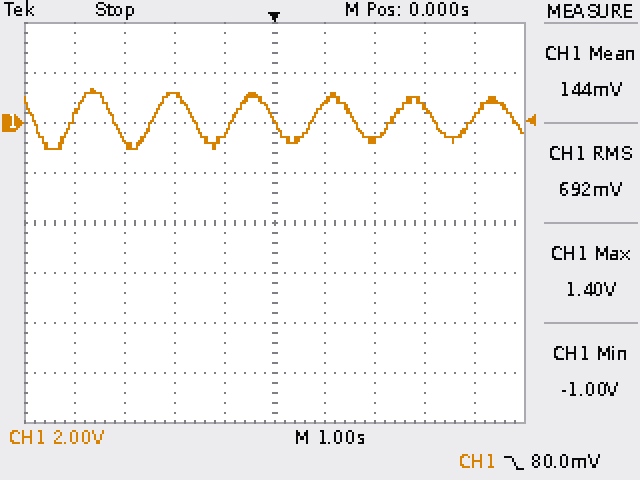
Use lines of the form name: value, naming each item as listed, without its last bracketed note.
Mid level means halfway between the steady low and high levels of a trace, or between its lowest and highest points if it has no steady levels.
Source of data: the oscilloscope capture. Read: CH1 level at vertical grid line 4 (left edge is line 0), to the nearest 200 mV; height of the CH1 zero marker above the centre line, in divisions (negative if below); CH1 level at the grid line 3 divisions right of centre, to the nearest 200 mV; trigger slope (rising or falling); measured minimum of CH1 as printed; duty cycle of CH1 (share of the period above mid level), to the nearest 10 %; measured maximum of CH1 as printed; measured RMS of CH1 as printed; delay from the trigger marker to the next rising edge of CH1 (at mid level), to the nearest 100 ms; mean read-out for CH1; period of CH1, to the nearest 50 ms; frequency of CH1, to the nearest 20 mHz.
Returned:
CH1 level at vertical grid line 4 (left edge is line 0), to the nearest 200 mV: -400 mV
height of the CH1 zero marker above the centre line, in divisions: +2.0 div
CH1 level at the grid line 3 divisions right of centre, to the nearest 200 mV: 600 mV
trigger slope: falling
measured minimum of CH1 as printed: -1.00 V
duty cycle of CH1 (share of the period above mid level), to the nearest 10 %: 50 %
measured maximum of CH1 as printed: 1.40 V
measured RMS of CH1 as printed: 692 mV
delay from the trigger marker to the next rising edge of CH1 (at mid level), to the nearest 100 ms: 800 ms
mean read-out for CH1: 144 mV
period of CH1, to the nearest 50 ms: 1.60 s
frequency of CH1, to the nearest 20 mHz: 620 mHz
